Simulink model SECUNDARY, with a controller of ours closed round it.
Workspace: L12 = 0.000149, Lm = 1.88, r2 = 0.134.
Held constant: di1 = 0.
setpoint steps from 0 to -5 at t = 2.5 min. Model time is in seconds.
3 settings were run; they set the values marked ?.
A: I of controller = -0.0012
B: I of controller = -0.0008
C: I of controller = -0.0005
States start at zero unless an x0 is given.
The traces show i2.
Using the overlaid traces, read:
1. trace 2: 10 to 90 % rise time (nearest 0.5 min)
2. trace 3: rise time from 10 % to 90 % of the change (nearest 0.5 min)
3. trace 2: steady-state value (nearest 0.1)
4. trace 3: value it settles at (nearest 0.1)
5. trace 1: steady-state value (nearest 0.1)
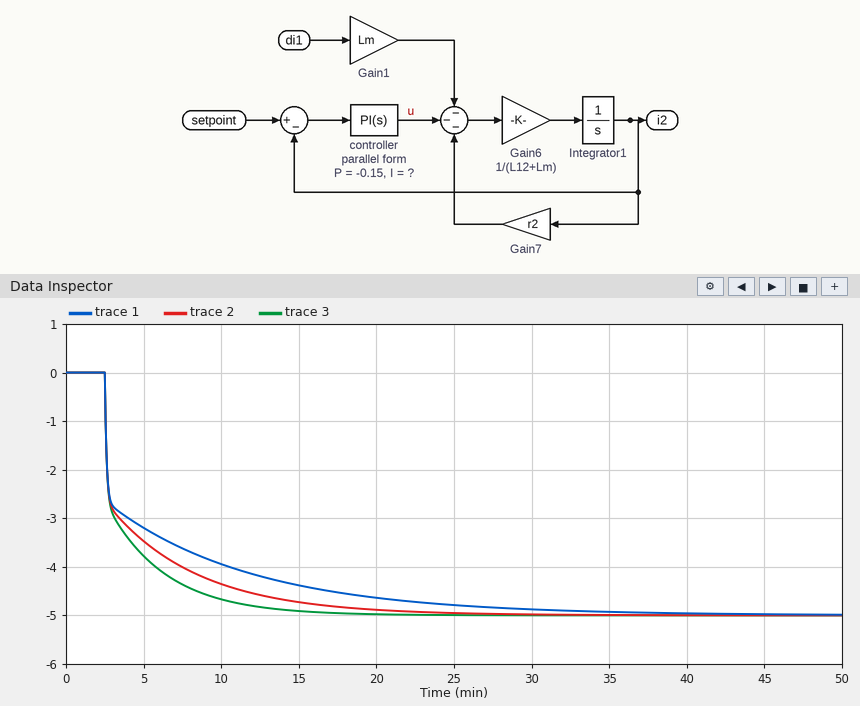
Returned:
9.0 min
6.0 min
-5.0
-5.0
-5.0
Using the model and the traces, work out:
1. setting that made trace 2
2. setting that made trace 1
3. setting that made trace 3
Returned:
B
C
A
